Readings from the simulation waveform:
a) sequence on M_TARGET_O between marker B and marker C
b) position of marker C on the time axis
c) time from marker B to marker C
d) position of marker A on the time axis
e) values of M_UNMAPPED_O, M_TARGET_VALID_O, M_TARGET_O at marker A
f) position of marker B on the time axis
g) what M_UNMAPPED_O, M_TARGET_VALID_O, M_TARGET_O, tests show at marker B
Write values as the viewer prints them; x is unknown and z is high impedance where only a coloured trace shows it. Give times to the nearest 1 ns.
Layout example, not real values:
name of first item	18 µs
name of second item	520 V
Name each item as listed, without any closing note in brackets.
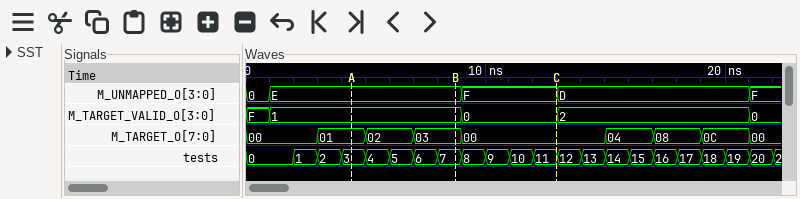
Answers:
sequence on M_TARGET_O between marker B and marker C	03, 00
position of marker C on the time axis	13 ns
time from marker B to marker C	4 ns
position of marker A on the time axis	4 ns
values of M_UNMAPPED_O, M_TARGET_VALID_O, M_TARGET_O at marker A	M_UNMAPPED_O=E, M_TARGET_VALID_O=1, M_TARGET_O=01
position of marker B on the time axis	9 ns
what M_UNMAPPED_O, M_TARGET_VALID_O, M_TARGET_O, tests show at marker B	M_UNMAPPED_O=E, M_TARGET_VALID_O=1, M_TARGET_O=03, tests=7
